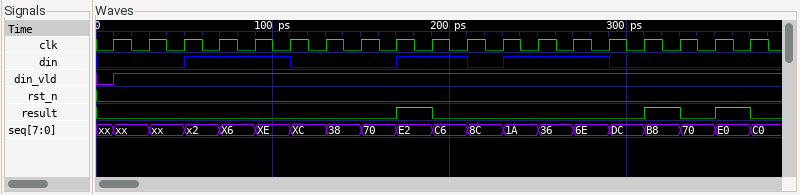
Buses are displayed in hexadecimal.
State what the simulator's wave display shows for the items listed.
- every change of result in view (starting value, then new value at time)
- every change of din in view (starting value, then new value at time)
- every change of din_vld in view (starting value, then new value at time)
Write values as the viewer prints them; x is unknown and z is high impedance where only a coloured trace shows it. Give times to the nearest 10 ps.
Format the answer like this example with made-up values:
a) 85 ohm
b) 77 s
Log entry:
a) 0, 1 at 170 ps, 0 at 190 ps, 1 at 310 ps, 0 at 330 ps, 1 at 350 ps, 0 at 370 ps
b) 0, 1 at 50 ps, 0 at 110 ps, 1 at 170 ps, 0 at 210 ps, 1 at 230 ps, 0 at 290 ps
c) 0, 1 at 10 ps
